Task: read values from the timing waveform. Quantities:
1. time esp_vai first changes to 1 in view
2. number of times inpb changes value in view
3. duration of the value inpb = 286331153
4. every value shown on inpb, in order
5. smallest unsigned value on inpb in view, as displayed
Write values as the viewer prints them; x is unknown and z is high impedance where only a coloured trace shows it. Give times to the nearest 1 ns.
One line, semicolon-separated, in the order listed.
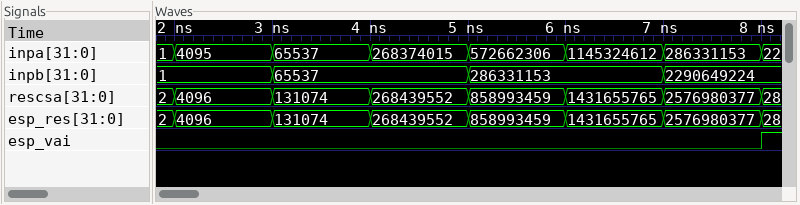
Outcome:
8 ns; 3; 2 ns; 1, 65537, 286331153, 2290649224; 1
